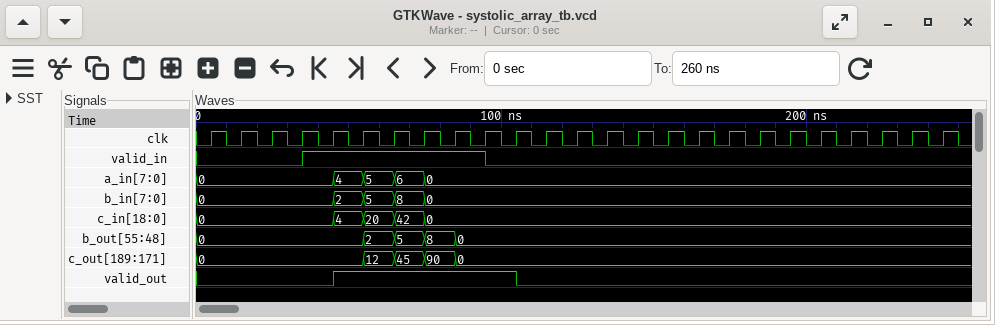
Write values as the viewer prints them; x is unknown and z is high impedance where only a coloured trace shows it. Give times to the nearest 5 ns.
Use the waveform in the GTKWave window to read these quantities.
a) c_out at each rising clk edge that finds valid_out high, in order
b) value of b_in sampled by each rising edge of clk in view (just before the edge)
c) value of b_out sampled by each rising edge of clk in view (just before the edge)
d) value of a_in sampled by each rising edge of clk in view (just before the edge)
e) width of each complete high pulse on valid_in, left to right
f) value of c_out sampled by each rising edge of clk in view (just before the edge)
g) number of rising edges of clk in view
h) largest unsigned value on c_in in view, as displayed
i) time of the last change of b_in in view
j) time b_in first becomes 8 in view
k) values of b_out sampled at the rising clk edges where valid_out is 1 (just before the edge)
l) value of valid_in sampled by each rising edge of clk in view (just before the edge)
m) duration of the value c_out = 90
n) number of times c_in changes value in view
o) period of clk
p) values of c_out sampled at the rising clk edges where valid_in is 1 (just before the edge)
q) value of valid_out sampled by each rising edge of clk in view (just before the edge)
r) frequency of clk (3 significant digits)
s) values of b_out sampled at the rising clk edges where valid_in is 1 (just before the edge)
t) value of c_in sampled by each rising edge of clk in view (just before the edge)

0, 12, 45, 90, 0, 0
0, 0, 0, 0, 0, 2, 5, 8, 0, 0, 0, 0, 0, 0, 0, 0, 0, 0, 0, 0, 0, 0, 0, 0, 0
0, 0, 0, 0, 0, 0, 2, 5, 8, 0, 0, 0, 0, 0, 0, 0, 0, 0, 0, 0, 0, 0, 0, 0, 0
0, 0, 0, 0, 0, 4, 5, 6, 0, 0, 0, 0, 0, 0, 0, 0, 0, 0, 0, 0, 0, 0, 0, 0, 0
60 ns
0, 0, 0, 0, 0, 0, 12, 45, 90, 0, 0, 0, 0, 0, 0, 0, 0, 0, 0, 0, 0, 0, 0, 0, 0
25
42
75 ns
65 ns
0, 2, 5, 8, 0, 0
0 0 0 0 1 1 1 1 1 1 0 0 0 0 0 0 0 0 0 0 0 0 0 0 0
10 ns
4
10 ns
0, 0, 12, 45, 90, 0
0 0 0 0 0 1 1 1 1 1 1 0 0 0 0 0 0 0 0 0 0 0 0 0 0
100 MHz
0, 0, 2, 5, 8, 0
0, 0, 0, 0, 0, 4, 20, 42, 0, 0, 0, 0, 0, 0, 0, 0, 0, 0, 0, 0, 0, 0, 0, 0, 0
